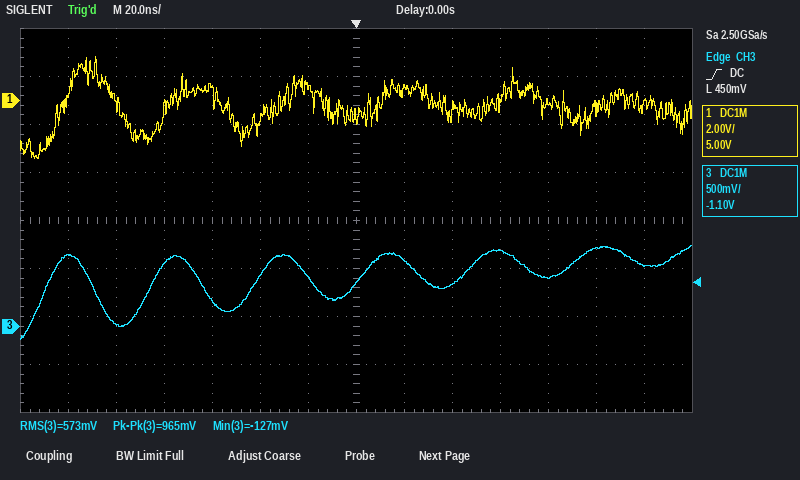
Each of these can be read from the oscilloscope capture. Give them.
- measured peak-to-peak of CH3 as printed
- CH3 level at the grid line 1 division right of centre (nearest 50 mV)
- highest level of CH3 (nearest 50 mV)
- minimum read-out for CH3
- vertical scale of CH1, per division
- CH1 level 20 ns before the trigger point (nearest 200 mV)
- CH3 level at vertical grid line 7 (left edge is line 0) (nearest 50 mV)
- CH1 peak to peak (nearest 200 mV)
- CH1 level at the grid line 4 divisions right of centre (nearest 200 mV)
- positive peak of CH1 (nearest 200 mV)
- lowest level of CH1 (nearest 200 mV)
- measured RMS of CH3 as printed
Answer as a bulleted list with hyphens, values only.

- 965 mV
- 700 mV
- 850 mV
- -127 mV
- 2 V
- 600 mV
- 450 mV
- 4.2 V
- 0.0 V
- 1.8 V
- -2.4 V
- 573 mV
